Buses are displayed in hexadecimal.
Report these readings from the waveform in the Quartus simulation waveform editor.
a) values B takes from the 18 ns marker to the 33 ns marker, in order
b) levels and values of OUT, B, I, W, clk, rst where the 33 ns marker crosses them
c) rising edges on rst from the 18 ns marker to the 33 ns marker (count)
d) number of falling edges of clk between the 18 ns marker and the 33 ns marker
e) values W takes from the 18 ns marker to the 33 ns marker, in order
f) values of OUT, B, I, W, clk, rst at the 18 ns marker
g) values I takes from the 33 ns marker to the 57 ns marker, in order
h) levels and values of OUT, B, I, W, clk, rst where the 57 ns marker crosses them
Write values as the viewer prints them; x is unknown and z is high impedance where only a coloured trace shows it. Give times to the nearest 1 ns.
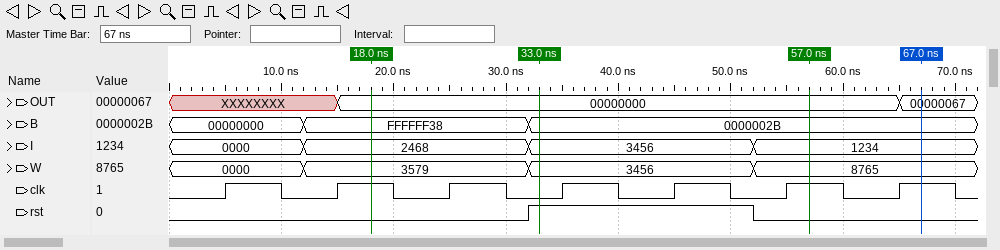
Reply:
FFFFFF38, 0000002B
OUT=00000000, B=0000002B, I=3456, W=3456, clk=0, rst=1
1
2
3579, 3456
OUT=00000000, B=FFFFFF38, I=2468, W=3579, clk=1, rst=0
3456, 1234
OUT=00000000, B=0000002B, I=1234, W=8765, clk=1, rst=0
